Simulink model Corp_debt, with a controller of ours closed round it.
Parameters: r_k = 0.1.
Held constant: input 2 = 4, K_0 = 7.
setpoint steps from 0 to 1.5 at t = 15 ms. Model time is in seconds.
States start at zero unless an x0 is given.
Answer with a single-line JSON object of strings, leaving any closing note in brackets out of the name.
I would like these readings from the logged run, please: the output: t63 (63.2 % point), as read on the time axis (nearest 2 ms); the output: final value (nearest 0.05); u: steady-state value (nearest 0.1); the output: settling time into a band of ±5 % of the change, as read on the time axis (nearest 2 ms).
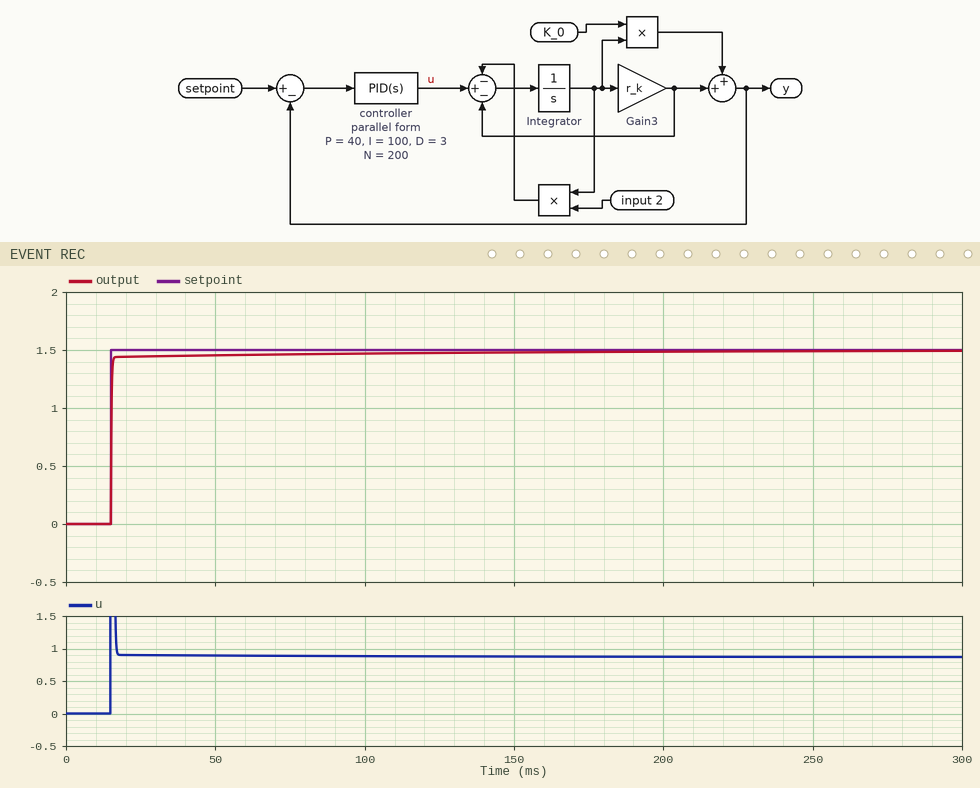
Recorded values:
{"the output: t63 (63.2 % point), as read on the time axis": "16 ms", "the output: final value": "1.50", "u: steady-state value": "0.9", "the output: settling time into a band of ±5 % of the change, as read on the time axis": "16 ms"}
